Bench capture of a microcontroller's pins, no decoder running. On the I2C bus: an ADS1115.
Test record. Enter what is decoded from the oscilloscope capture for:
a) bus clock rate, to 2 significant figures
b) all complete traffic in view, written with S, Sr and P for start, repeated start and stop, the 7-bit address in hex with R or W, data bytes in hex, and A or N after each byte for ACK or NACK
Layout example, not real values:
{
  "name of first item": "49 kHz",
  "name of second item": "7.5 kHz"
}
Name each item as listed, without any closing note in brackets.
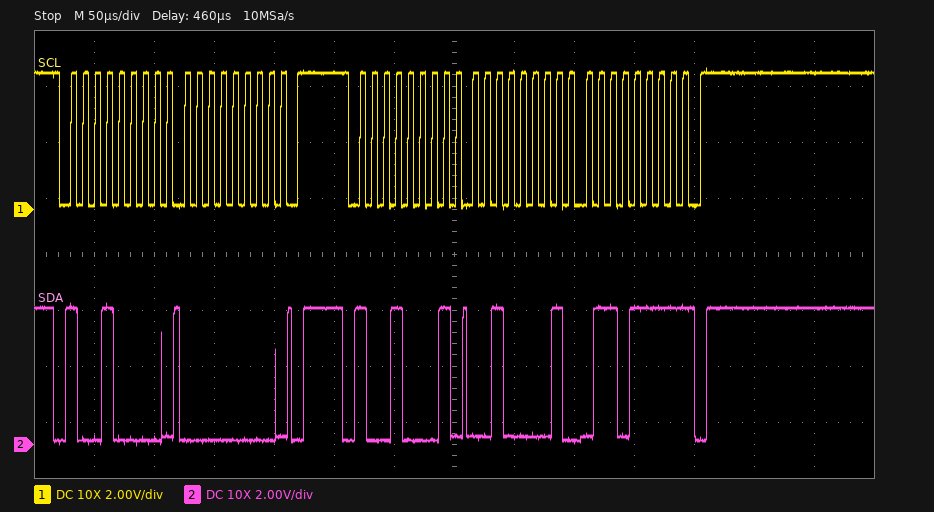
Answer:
{
  "bus clock rate, to 2 significant figures": "100 kHz",
  "all complete traffic in view, written with S, Sr and P for start, repeated start and stop, the 7-bit address in hex with R or W, data bytes in hex, and A or N after each byte for ACK or NACK": "S 48W A 00 A P S 48R A 21 A 6F N P"
}
